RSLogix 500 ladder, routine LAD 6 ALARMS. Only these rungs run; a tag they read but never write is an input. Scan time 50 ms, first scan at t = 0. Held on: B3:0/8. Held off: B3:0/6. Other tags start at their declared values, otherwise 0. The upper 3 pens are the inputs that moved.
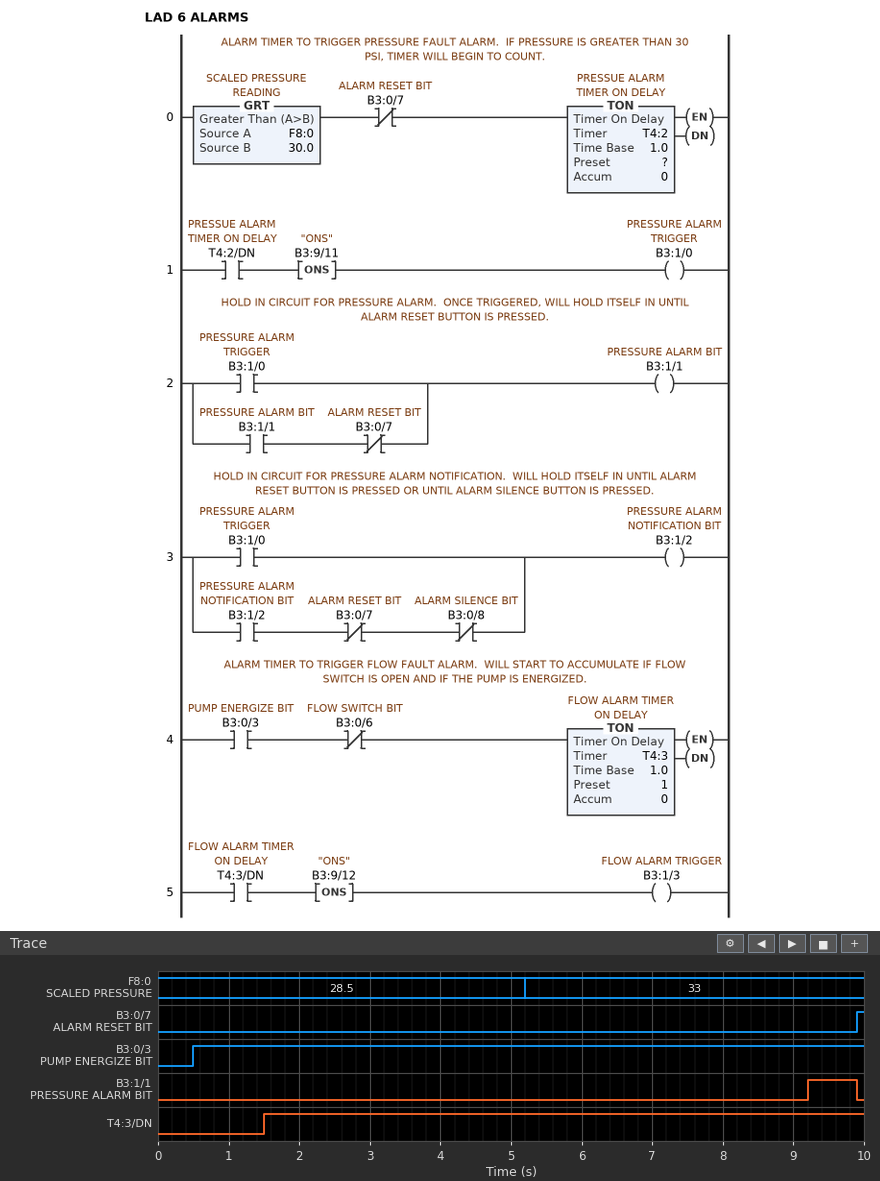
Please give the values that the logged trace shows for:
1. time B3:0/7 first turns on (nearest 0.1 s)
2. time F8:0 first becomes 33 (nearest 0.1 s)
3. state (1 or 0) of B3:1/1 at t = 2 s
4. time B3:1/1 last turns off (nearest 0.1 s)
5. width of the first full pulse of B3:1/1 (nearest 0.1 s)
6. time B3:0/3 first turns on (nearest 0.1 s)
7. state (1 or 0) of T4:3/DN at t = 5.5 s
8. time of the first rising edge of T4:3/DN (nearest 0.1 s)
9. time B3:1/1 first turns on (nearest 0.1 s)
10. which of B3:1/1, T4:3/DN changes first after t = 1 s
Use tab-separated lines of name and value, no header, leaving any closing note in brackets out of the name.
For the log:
time B3:0/7 first turns on	9.9 s
time F8:0 first becomes 33	5.2 s
state (1 or 0) of B3:1/1 at t = 2 s	0
time B3:1/1 last turns off	9.9 s
width of the first full pulse of B3:1/1	0.7 s
time B3:0/3 first turns on	0.5 s
state (1 or 0) of T4:3/DN at t = 5.5 s	1
time of the first rising edge of T4:3/DN	1.5 s
time B3:1/1 first turns on	9.2 s
which of B3:1/1, T4:3/DN changes first after t = 1 s	T4:3/DN
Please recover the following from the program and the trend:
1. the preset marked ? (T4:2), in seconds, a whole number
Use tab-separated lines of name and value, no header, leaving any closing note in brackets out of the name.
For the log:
the preset marked ? (T4:2), in seconds, a whole number	4 s
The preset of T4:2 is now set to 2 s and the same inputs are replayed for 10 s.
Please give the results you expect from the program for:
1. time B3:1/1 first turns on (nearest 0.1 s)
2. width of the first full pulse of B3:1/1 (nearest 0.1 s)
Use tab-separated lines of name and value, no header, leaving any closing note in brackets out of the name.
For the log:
time B3:1/1 first turns on	7.2 s
width of the first full pulse of B3:1/1	2.7 s
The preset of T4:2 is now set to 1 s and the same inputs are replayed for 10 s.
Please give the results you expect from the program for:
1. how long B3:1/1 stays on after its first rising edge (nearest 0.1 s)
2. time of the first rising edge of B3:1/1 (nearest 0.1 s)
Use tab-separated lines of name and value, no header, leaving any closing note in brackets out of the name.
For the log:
how long B3:1/1 stays on after its first rising edge	3.7 s
time of the first rising edge of B3:1/1	6.2 s
